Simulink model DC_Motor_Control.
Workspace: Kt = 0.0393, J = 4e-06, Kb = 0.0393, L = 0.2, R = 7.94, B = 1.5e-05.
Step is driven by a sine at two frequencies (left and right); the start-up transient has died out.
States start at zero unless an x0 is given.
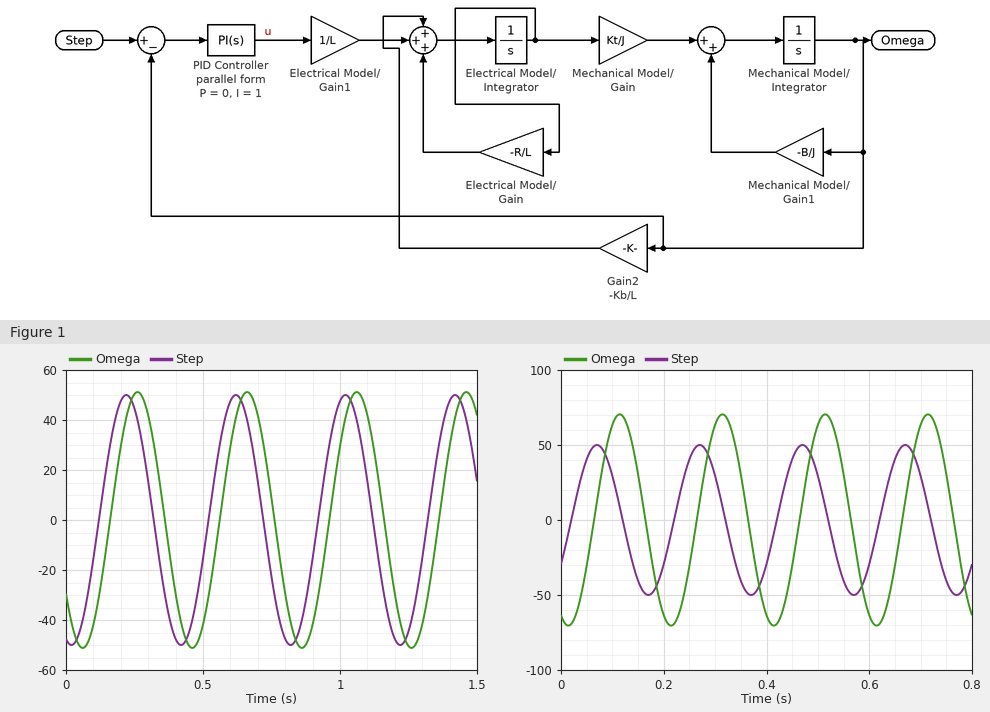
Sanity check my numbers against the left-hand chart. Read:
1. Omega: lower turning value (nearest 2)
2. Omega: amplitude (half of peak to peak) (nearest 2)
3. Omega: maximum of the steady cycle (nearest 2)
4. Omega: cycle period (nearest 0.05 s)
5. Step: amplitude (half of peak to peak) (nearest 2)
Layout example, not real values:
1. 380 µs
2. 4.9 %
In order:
1. -52
2. 52
3. 52
4. 0.40 s
5. 50
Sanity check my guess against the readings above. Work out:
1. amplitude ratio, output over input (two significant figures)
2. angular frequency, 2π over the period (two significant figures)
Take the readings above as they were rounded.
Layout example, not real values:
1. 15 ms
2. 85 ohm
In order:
1. 1.0
2. 16 rad/s
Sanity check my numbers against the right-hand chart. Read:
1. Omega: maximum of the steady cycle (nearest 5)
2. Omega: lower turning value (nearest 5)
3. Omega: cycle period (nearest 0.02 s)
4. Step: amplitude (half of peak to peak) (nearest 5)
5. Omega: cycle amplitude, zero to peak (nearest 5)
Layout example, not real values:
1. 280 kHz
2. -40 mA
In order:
1. 70
2. -70
3. 0.20 s
4. 50
5. 70
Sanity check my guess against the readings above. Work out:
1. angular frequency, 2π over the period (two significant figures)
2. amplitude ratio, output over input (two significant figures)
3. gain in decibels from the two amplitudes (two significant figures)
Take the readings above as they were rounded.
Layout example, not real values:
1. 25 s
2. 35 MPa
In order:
1. 31 rad/s
2. 1.4
3. 2.9 dB
